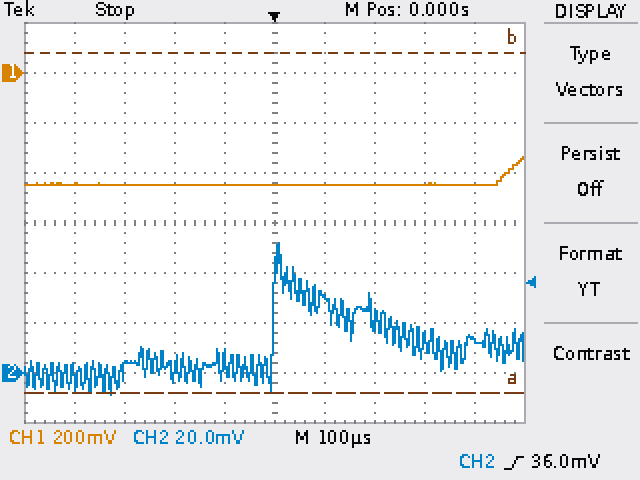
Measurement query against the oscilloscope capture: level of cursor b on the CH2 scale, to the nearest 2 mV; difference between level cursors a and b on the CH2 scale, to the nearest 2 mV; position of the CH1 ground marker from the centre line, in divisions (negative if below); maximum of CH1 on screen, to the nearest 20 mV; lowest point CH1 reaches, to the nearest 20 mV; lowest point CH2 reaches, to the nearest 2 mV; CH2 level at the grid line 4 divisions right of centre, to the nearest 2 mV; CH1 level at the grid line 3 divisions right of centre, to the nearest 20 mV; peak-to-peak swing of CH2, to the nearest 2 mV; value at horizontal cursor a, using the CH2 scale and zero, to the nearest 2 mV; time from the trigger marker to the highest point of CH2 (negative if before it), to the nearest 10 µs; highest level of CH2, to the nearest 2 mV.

128 mV
136 mV
+3.0 div
-340 mV
-440 mV
-8 mV
14 mV
-440 mV
60 mV
-8 mV
+10 µs
52 mV
